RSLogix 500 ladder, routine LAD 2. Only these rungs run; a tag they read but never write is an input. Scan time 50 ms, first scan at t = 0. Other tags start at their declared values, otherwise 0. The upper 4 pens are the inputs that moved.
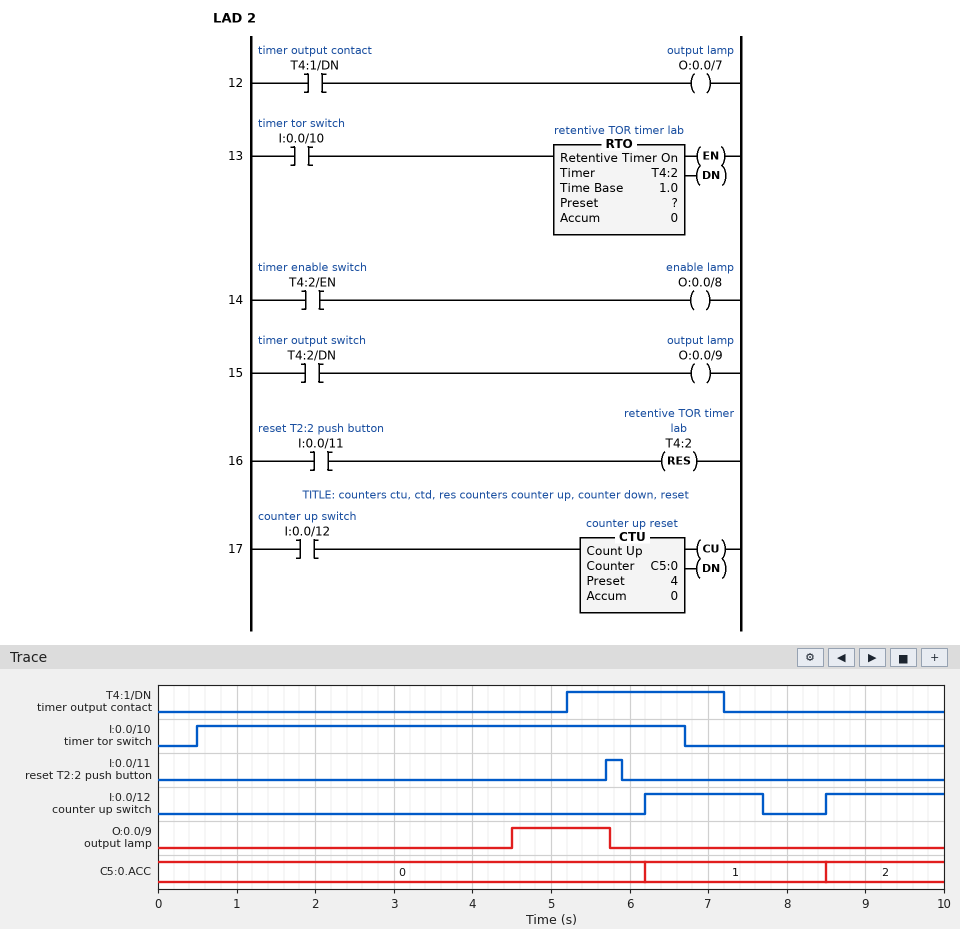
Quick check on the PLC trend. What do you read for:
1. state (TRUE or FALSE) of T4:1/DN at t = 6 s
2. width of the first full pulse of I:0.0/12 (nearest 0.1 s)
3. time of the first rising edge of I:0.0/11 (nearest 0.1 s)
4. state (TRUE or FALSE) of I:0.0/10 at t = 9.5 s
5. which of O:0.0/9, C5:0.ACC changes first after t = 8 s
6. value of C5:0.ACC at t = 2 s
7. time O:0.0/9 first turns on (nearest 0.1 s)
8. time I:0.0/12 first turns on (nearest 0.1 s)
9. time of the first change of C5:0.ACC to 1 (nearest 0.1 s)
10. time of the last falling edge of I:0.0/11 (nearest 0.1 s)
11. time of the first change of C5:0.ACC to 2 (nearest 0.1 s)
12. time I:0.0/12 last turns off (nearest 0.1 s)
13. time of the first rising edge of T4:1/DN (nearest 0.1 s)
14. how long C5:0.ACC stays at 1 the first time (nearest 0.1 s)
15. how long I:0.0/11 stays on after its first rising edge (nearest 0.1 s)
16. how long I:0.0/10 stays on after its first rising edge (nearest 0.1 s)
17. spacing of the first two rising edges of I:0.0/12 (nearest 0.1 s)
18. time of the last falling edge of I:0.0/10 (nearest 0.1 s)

TRUE
1.5 s
5.7 s
FALSE
C5:0.ACC
0
4.5 s
6.2 s
6.2 s
5.9 s
8.5 s
7.7 s
5.2 s
2.3 s
0.2 s
6.2 s
2.3 s
6.7 s
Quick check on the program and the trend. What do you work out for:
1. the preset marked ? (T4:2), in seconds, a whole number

4 s
